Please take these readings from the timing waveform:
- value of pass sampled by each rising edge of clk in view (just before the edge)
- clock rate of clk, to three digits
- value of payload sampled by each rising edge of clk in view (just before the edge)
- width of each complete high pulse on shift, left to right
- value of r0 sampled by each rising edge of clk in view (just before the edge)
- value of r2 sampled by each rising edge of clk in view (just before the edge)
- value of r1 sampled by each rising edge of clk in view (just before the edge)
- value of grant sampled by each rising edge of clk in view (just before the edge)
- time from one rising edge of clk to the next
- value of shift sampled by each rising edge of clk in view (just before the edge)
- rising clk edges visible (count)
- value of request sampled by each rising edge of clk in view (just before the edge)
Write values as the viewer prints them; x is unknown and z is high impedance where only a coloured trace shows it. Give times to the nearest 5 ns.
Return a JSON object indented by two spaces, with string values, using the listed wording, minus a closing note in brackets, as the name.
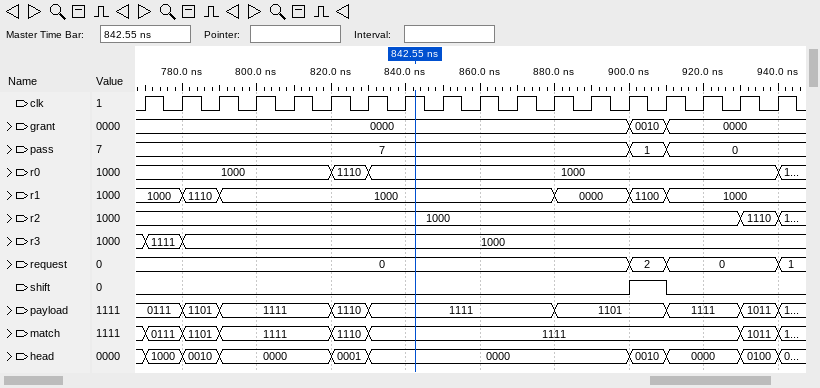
{
  "value of pass sampled by each rising edge of clk in view": "7, 7, 7, 7, 7, 7, 7, 7, 7, 7, 7, 7, 7, 7, 1, 0, 0, 0",
  "clock rate of clk, to three digits": "100 MHz",
  "value of payload sampled by each rising edge of clk in view": "0111, 0111, 1101, 1111, 1111, 1111, 1110, 1111, 1111, 1111, 1111, 1111, 1101, 1101, 1101, 1111, 1111, 1011",
  "width of each complete high pulse on shift, left to right": "10 ns",
  "value of r0 sampled by each rising edge of clk in view": "1000, 1000, 1000, 1000, 1000, 1000, 1110, 1000, 1000, 1000, 1000, 1000, 1000, 1000, 1000, 1000, 1000, 1000",
  "value of r2 sampled by each rising edge of clk in view": "1000, 1000, 1000, 1000, 1000, 1000, 1000, 1000, 1000, 1000, 1000, 1000, 1000, 1000, 1000, 1000, 1000, 1110",
  "value of r1 sampled by each rising edge of clk in view": "1000, 1000, 1110, 1000, 1000, 1000, 1000, 1000, 1000, 1000, 1000, 1000, 0000, 0000, 1100, 1000, 1000, 1000",
  "value of grant sampled by each rising edge of clk in view": "0000, 0000, 0000, 0000, 0000, 0000, 0000, 0000, 0000, 0000, 0000, 0000, 0000, 0000, 0010, 0000, 0000, 0000",
  "time from one rising edge of clk to the next": "10 ns",
  "value of shift sampled by each rising edge of clk in view": "0 0 0 0 0 0 0 0 0 0 0 0 0 0 1 0 0 0",
  "rising clk edges visible": "18",
  "value of request sampled by each rising edge of clk in view": "0, 0, 0, 0, 0, 0, 0, 0, 0, 0, 0, 0, 0, 0, 2, 0, 0, 0"
}
